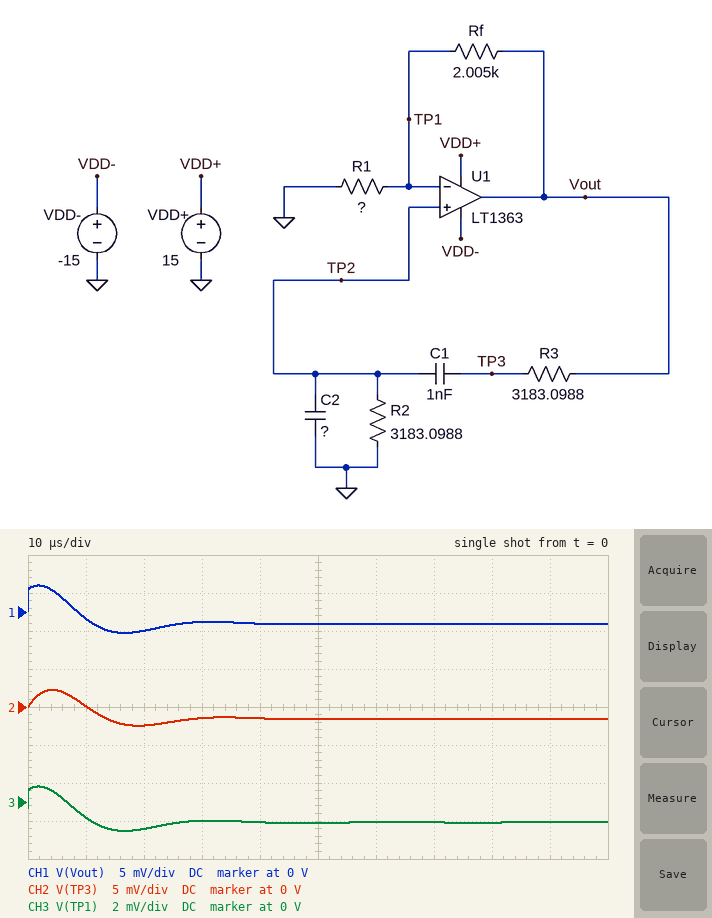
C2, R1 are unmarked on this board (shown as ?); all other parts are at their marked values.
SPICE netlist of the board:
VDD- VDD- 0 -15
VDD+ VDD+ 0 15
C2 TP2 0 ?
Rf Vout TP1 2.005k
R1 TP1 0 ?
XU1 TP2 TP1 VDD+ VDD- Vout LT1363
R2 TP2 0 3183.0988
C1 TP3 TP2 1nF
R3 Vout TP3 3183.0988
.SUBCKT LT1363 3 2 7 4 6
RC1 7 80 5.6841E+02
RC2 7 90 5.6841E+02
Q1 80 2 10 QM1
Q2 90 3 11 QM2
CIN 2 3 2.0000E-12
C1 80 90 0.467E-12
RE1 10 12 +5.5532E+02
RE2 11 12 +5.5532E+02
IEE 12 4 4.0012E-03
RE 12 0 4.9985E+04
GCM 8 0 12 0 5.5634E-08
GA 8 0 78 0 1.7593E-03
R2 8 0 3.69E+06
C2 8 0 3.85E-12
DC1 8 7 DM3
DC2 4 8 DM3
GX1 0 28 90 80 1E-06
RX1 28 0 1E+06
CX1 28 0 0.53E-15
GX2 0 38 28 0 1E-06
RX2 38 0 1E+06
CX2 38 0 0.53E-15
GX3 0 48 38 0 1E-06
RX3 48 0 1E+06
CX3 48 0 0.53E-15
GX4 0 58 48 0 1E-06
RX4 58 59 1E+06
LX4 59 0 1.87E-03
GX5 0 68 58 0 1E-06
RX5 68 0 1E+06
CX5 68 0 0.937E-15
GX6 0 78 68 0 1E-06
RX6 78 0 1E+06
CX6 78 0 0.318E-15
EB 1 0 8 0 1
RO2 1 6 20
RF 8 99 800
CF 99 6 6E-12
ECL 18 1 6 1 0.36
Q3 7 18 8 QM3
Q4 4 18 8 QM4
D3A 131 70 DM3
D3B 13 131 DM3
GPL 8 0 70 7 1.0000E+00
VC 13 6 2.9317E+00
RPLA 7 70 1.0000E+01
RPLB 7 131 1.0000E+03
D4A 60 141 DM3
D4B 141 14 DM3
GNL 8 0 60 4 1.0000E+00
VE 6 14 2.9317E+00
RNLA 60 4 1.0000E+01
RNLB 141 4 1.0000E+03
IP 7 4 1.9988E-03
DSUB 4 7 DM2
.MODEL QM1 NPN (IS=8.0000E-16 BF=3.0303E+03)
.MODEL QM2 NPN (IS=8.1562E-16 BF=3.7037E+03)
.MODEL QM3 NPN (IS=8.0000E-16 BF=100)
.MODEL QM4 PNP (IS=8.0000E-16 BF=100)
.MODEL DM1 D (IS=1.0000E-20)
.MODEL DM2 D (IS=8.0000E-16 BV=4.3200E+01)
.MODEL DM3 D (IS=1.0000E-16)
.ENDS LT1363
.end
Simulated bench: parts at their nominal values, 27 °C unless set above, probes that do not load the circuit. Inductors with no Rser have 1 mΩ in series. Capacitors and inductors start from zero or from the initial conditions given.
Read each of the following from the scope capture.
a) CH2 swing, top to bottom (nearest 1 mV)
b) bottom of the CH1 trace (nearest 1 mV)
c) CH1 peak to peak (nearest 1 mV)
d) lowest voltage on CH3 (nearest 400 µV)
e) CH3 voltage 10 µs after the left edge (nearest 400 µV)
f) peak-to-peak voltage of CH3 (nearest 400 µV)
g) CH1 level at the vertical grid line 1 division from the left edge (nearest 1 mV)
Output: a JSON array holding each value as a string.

["5 mV", "-3 mV", "6 mV", "-1.6 mV", "-800 µV", "2.4 mV", "-1 mV"]
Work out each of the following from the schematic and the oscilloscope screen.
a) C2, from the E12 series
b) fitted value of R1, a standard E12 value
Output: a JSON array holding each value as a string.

["1.8 nF", "1.2 kΩ"]
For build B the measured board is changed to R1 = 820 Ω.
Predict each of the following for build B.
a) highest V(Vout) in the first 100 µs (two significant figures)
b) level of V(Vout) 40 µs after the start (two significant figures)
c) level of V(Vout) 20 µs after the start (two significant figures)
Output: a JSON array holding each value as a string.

["4.8 mV", "-3.8 mV", "-5.5 mV"]
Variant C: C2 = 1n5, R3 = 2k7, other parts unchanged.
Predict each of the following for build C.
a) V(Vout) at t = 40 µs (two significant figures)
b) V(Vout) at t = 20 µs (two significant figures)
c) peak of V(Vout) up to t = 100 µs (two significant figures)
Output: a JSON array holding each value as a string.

["-1.8 mV", "-1.9 mV", "4.0 mV"]
